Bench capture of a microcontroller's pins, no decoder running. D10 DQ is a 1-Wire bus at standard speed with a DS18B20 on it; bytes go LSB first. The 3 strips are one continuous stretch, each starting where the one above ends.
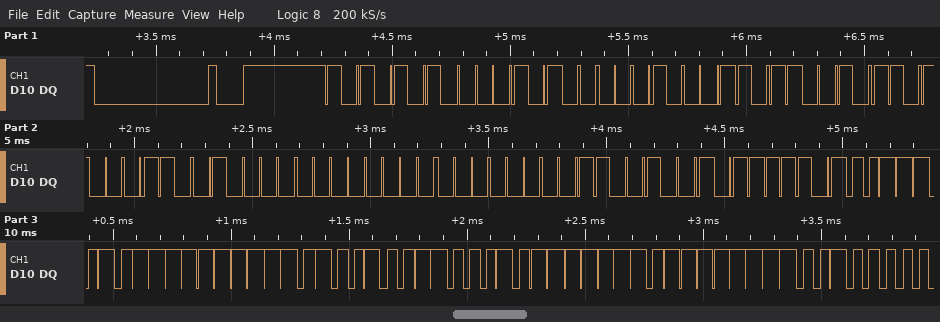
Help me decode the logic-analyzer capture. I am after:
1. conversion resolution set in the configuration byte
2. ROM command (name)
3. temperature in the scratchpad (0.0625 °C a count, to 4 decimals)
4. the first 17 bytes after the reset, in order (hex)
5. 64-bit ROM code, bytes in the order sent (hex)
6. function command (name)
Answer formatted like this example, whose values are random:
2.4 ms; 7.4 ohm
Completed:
12 bits; Match ROM; -10.2500 °C; 55 28 88 4D 8B 09 00 00 93 BE 5C FF 4B 46 7F FF 04; 28 88 4D 8B 09 00 00 93; Read Scratchpad
